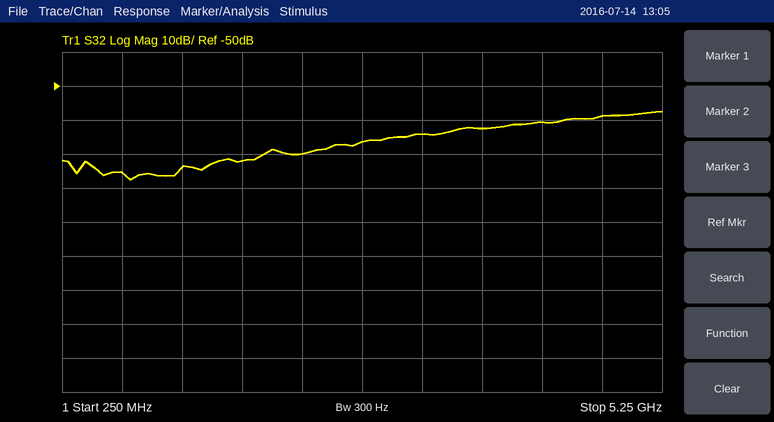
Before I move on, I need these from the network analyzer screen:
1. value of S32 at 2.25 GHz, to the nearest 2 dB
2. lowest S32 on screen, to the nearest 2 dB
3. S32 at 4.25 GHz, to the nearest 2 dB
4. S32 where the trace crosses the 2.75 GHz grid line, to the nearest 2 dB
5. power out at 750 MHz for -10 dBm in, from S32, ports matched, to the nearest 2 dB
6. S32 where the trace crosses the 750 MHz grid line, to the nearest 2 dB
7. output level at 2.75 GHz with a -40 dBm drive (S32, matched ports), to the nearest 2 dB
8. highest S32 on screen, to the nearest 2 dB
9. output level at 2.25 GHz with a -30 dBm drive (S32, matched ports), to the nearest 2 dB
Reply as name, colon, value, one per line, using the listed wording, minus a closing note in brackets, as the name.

value of S32 at 2.25 GHz, to the nearest 2 dB: -70 dB
lowest S32 on screen, to the nearest 2 dB: -78 dB
S32 at 4.25 GHz, to the nearest 2 dB: -60 dB
S32 where the trace crosses the 2.75 GHz grid line, to the nearest 2 dB: -66 dB
power out at 750 MHz for -10 dBm in, from S32, ports matched, to the nearest 2 dB: -86 dBm
S32 where the trace crosses the 750 MHz grid line, to the nearest 2 dB: -76 dB
output level at 2.75 GHz with a -40 dBm drive (S32, matched ports), to the nearest 2 dB: -106 dBm
highest S32 on screen, to the nearest 2 dB: -58 dB
output level at 2.25 GHz with a -30 dBm drive (S32, matched ports), to the nearest 2 dB: -100 dBm
